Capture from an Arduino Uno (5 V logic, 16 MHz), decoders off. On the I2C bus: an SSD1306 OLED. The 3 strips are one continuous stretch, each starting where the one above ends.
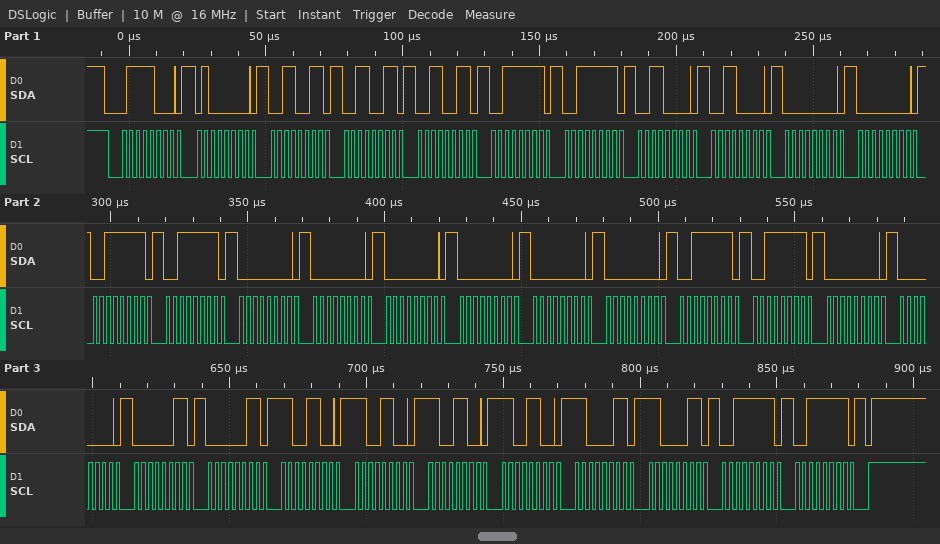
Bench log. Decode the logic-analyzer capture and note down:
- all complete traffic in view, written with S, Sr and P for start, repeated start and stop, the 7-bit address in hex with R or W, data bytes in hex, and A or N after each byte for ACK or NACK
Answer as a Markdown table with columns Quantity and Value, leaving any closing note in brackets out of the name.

| Quantity | Value |
|---|---|
| all complete traffic in view, written with S, Sr and P for start, repeated start and stop, the 7-bit address in hex with R or W, data bytes in hex, and A or N after each byte for ACK or NACK | S 3CW A 40 A 33 A 33 A 33 A 3F A 3F A 30 A 30 A 00 A 00 A 3F A 3F A 00 A 00 A 00 A 00 A 00 A 00 A 3F A 3F A 00 A 00 A 03 A 03 A CC A CC A CC A CC A C3 A C3 A 3F A 3F A P |
